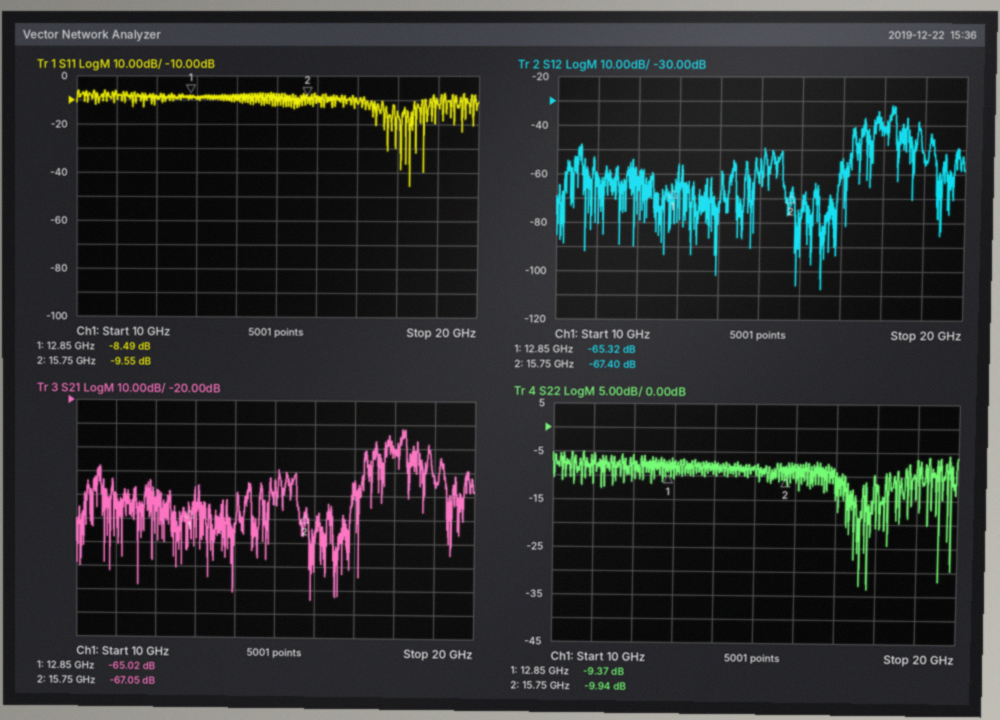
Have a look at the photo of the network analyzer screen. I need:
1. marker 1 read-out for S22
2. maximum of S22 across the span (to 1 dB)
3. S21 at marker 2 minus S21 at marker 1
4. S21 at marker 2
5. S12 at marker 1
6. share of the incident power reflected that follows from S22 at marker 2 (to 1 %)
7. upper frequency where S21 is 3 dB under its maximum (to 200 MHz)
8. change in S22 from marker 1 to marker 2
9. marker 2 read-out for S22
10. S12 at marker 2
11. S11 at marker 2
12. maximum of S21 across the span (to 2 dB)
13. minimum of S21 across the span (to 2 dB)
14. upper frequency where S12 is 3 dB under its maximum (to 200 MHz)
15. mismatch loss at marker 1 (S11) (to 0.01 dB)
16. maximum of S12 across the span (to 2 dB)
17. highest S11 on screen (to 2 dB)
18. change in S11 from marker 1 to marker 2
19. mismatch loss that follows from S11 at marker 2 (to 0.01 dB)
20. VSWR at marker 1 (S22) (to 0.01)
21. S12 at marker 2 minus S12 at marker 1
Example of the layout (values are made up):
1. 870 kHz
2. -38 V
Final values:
1. -9.37 dB
2. -5 dB
3. -2.03 dB
4. -67.05 dB
5. -65.32 dB
6. 10 %
7. 18.2 GHz
8. -0.57 dB
9. -9.94 dB
10. -67.40 dB
11. -9.55 dB
12. -32 dB
13. -104 dB
14. 18.2 GHz
15. 0.66 dB
16. -32 dB
17. -6 dB
18. -1.06 dB
19. 0.51 dB
20. 2.03
21. -2.08 dB
